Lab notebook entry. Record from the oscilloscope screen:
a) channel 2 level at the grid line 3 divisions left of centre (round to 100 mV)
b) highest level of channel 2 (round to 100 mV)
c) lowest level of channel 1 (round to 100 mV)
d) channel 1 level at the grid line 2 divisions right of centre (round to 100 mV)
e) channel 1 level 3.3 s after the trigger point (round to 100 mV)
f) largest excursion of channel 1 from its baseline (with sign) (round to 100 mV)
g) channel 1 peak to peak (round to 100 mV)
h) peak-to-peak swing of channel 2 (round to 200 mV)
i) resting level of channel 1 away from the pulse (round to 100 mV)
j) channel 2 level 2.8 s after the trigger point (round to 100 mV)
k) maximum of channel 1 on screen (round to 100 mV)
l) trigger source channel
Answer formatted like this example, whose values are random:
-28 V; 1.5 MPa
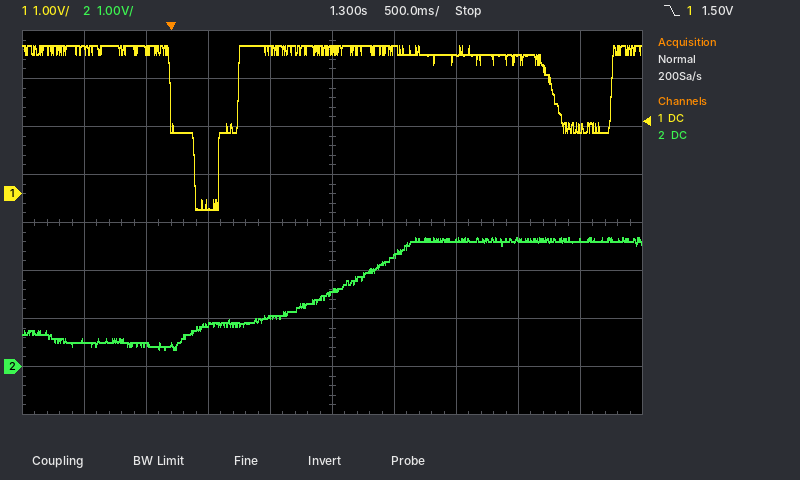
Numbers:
500 mV; 2.7 V; -300 mV; 2.9 V; 1.4 V; -3.3 V; 3.4 V; 2.4 V; 3.0 V; 2.6 V; 3.1 V; channel 1
